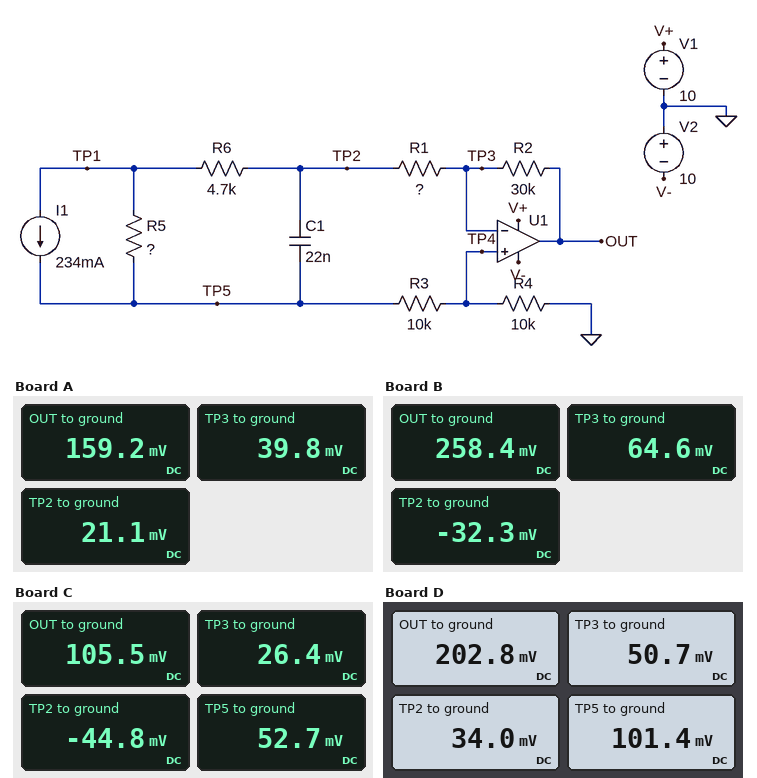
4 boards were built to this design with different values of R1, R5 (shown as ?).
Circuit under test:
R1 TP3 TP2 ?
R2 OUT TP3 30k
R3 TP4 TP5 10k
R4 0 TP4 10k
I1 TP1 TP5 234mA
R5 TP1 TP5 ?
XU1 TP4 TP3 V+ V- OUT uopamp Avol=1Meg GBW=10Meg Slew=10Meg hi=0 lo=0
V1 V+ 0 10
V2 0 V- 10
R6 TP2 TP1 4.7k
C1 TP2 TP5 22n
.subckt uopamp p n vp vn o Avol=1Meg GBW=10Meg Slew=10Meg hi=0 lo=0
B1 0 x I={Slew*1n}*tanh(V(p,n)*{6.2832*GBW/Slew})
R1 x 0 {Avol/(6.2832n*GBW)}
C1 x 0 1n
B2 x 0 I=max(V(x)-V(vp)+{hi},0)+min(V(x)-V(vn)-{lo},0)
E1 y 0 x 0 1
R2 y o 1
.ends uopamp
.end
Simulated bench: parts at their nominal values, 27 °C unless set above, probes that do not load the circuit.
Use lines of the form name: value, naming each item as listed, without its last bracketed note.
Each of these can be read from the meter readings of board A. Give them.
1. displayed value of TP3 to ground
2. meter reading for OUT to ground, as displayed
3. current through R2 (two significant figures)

displayed value of TP3 to ground: 39.8 mV
meter reading for OUT to ground, as displayed: 159.2 mV
current through R2: 4.0 µA
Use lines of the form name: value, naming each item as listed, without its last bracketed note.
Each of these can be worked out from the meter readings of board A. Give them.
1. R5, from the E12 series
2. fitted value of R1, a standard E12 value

R5, from the E12 series: 0.33 Ω
fitted value of R1, a standard E12 value: 4.7 kΩ
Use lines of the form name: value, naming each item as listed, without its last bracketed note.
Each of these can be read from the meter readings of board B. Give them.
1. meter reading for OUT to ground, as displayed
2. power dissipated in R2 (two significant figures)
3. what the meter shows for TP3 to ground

meter reading for OUT to ground, as displayed: 258.4 mV
power dissipated in R2: 1.3 µW
what the meter shows for TP3 to ground: 64.6 mV
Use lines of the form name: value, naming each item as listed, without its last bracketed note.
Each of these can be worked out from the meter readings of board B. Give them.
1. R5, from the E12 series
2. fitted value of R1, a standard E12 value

R5, from the E12 series: 0.82 Ω
fitted value of R1, a standard E12 value: 15 kΩ
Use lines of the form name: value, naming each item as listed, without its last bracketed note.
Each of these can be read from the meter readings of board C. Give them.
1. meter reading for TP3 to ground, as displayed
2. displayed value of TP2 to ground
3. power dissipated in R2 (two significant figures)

meter reading for TP3 to ground, as displayed: 26.4 mV
displayed value of TP2 to ground: -44.8 mV
power dissipated in R2: 210 nW
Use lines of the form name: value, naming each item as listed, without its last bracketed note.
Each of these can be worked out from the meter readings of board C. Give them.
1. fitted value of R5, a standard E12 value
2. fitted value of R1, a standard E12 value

fitted value of R5, a standard E12 value: 0.47 Ω
fitted value of R1, a standard E12 value: 27 kΩ
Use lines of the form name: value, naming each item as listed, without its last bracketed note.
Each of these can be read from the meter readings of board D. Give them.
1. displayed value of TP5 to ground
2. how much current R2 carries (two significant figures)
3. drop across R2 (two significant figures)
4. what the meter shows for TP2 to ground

displayed value of TP5 to ground: 101.4 mV
how much current R2 carries: 5.1 µA
drop across R2: 150 mV
what the meter shows for TP2 to ground: 34.0 mV
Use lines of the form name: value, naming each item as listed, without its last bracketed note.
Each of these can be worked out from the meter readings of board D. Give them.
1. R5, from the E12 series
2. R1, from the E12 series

R5, from the E12 series: 0.39 Ω
R1, from the E12 series: 3.3 kΩ
